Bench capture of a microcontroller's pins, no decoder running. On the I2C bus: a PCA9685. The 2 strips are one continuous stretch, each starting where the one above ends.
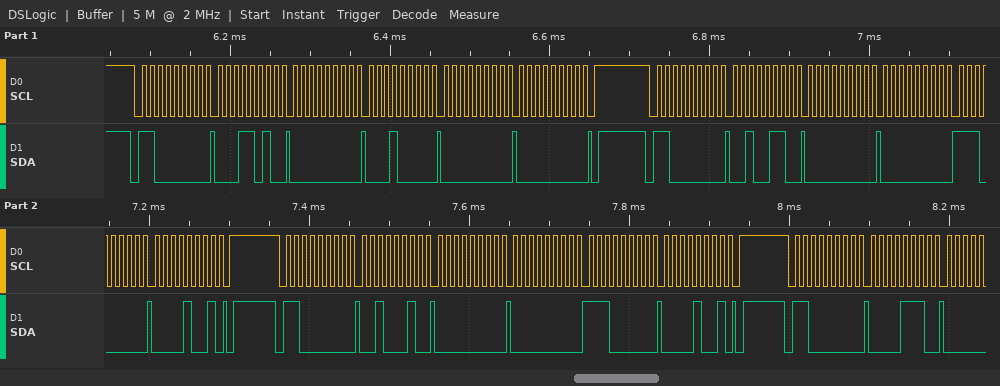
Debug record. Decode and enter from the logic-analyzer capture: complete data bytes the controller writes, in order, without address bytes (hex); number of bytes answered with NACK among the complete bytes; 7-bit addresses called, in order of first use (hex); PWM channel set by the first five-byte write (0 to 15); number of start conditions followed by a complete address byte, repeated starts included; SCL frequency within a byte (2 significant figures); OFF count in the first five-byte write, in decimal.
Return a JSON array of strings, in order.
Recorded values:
["1A 00 10 00 00 26 00 00 E0 09 22 00 00 E0 09 0E", "0", "0x60", "5", "4", "100 kHz", "0"]
